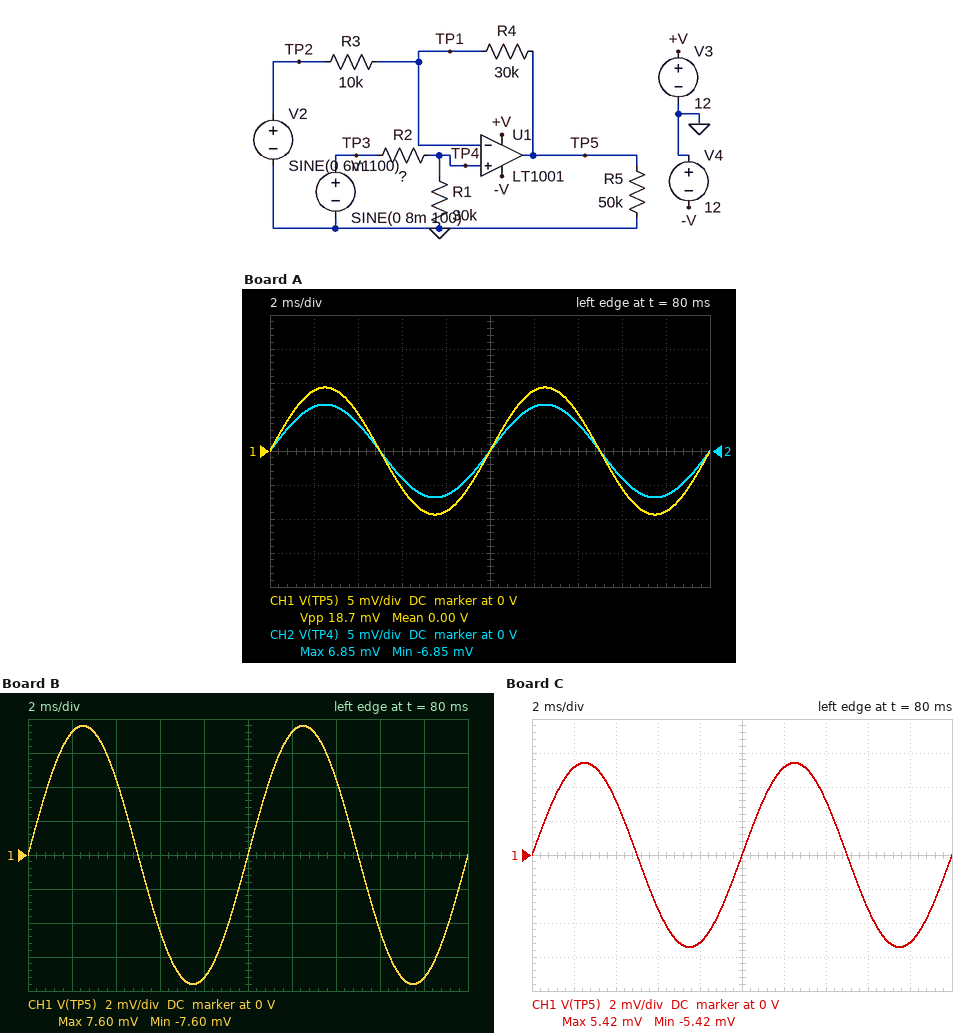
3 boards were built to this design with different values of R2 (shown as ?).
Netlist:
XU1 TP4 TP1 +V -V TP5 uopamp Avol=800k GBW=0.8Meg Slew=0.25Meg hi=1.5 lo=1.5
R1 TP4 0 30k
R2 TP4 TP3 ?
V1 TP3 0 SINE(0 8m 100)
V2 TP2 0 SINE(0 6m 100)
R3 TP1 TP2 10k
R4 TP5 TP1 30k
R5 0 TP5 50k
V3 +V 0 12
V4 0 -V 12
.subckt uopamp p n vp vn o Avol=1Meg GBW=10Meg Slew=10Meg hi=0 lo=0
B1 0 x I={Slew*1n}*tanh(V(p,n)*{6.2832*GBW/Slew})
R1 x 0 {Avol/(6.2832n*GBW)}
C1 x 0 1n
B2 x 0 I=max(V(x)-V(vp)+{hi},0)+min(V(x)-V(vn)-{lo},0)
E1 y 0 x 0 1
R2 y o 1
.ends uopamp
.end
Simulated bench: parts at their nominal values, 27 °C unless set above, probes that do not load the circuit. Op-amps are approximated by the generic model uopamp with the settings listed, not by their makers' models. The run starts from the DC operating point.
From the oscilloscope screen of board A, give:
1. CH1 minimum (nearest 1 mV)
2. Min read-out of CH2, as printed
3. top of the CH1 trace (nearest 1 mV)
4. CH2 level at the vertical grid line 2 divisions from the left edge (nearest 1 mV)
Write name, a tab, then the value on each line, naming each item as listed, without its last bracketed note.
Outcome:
CH1 minimum	-9 mV
Min read-out of CH2, as printed	-6.85 mV
top of the CH1 trace	9 mV
CH2 level at the vertical grid line 2 divisions from the left edge	4 mV
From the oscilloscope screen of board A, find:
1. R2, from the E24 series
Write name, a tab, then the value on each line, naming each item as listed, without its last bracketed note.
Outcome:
R2, from the E24 series	5.1 kΩ
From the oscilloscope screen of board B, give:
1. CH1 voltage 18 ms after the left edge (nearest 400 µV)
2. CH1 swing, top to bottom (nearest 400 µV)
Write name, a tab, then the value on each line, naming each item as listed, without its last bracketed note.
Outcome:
CH1 voltage 18 ms after the left edge	-7.2 mV
CH1 swing, top to bottom	15.2 mV
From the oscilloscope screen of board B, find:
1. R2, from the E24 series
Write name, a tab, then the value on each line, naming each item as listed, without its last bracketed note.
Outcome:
R2, from the E24 series	7.5 kΩ
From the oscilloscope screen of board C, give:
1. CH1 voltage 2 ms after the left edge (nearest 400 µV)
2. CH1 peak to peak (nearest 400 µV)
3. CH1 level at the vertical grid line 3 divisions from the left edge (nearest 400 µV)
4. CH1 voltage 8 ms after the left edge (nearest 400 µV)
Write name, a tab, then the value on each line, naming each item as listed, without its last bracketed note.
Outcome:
CH1 voltage 2 ms after the left edge	5.2 mV
CH1 peak to peak	10.8 mV
CH1 level at the vertical grid line 3 divisions from the left edge	-3.2 mV
CH1 voltage 8 ms after the left edge	-5.2 mV
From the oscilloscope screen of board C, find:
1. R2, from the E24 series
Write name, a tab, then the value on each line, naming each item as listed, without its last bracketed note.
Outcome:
R2, from the E24 series	11 kΩ
